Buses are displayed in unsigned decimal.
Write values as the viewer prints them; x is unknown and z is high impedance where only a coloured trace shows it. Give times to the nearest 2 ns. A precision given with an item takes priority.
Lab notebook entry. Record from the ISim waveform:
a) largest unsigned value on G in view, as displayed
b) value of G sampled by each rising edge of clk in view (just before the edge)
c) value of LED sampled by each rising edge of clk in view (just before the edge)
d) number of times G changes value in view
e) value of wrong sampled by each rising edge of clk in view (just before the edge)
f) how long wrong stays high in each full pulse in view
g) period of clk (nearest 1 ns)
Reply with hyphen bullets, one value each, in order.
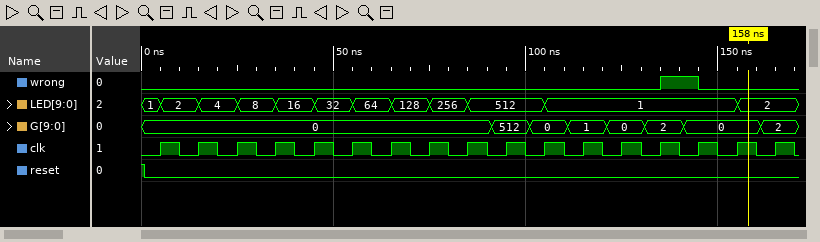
- 512
- 0, 0, 0, 0, 0, 0, 0, 0, 0, 512, 0, 1, 0, 2, 0, 0, 2
- 1, 2, 4, 8, 16, 32, 64, 128, 256, 512, 512, 1, 1, 1, 1, 1, 2
- 7
- 0 0 0 0 0 0 0 0 0 0 0 0 0 0 1 0 0
- 10 ns
- 10 ns
